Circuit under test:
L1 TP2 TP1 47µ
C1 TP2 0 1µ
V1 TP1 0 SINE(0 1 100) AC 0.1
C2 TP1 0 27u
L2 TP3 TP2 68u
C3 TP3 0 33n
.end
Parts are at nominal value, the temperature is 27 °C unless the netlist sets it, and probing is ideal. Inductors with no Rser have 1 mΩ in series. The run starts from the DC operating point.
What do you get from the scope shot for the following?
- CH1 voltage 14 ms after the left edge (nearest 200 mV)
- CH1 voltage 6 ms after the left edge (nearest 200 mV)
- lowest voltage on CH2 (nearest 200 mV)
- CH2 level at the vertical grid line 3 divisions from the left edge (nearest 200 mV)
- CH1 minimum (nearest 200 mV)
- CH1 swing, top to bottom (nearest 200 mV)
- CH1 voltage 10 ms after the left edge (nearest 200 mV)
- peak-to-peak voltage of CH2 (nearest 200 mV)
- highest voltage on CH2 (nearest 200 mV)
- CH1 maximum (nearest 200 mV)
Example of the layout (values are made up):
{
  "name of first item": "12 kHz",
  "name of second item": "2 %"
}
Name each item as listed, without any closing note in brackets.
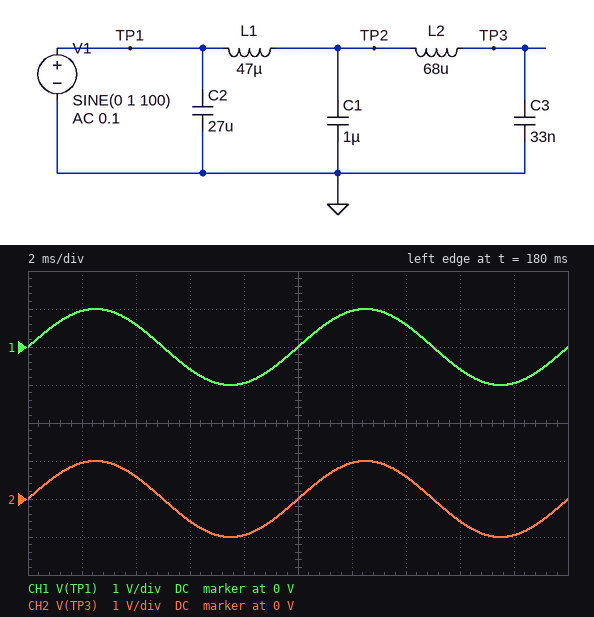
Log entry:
{
  "CH1 voltage 14 ms after the left edge": "600 mV",
  "CH1 voltage 6 ms after the left edge": "-600 mV",
  "lowest voltage on CH2": "-1.0 V",
  "CH2 level at the vertical grid line 3 divisions from the left edge": "-600 mV",
  "CH1 minimum": "-1.0 V",
  "CH1 swing, top to bottom": "2.0 V",
  "CH1 voltage 10 ms after the left edge": "0 V",
  "peak-to-peak voltage of CH2": "2.0 V",
  "highest voltage on CH2": "1.0 V",
  "CH1 maximum": "1.0 V"
}
